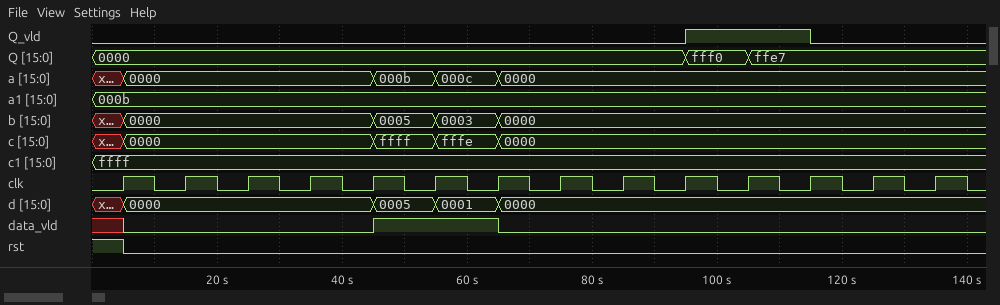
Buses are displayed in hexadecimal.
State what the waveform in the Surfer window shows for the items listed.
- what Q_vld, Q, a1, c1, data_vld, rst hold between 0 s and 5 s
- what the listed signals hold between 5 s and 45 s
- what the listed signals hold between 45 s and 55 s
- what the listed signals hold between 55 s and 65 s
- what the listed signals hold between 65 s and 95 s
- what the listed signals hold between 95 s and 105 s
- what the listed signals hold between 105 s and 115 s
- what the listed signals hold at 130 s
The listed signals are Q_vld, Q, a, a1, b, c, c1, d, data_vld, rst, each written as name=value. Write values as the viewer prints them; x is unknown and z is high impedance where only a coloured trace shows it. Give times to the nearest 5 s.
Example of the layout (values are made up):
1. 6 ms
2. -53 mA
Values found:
1. Q_vld=0, Q=0000, a1=000b, c1=ffff, data_vld=x, rst=1
2. Q_vld=0, Q=0000, a=0000, a1=000b, b=0000, c=0000, c1=ffff, d=0000, data_vld=0, rst=0
3. Q_vld=0, Q=0000, a=000b, a1=000b, b=0005, c=ffff, c1=ffff, d=0005, data_vld=1, rst=0
4. Q_vld=0, Q=0000, a=000c, a1=000b, b=0003, c=fffe, c1=ffff, d=0001, data_vld=1, rst=0
5. Q_vld=0, Q=0000, a=0000, a1=000b, b=0000, c=0000, c1=ffff, d=0000, data_vld=0, rst=0
6. Q_vld=1, Q=fff0, a=0000, a1=000b, b=0000, c=0000, c1=ffff, d=0000, data_vld=0, rst=0
7. Q_vld=1, Q=ffe7, a=0000, a1=000b, b=0000, c=0000, c1=ffff, d=0000, data_vld=0, rst=0
8. Q_vld=0, Q=ffe7, a=0000, a1=000b, b=0000, c=0000, c1=ffff, d=0000, data_vld=0, rst=0
